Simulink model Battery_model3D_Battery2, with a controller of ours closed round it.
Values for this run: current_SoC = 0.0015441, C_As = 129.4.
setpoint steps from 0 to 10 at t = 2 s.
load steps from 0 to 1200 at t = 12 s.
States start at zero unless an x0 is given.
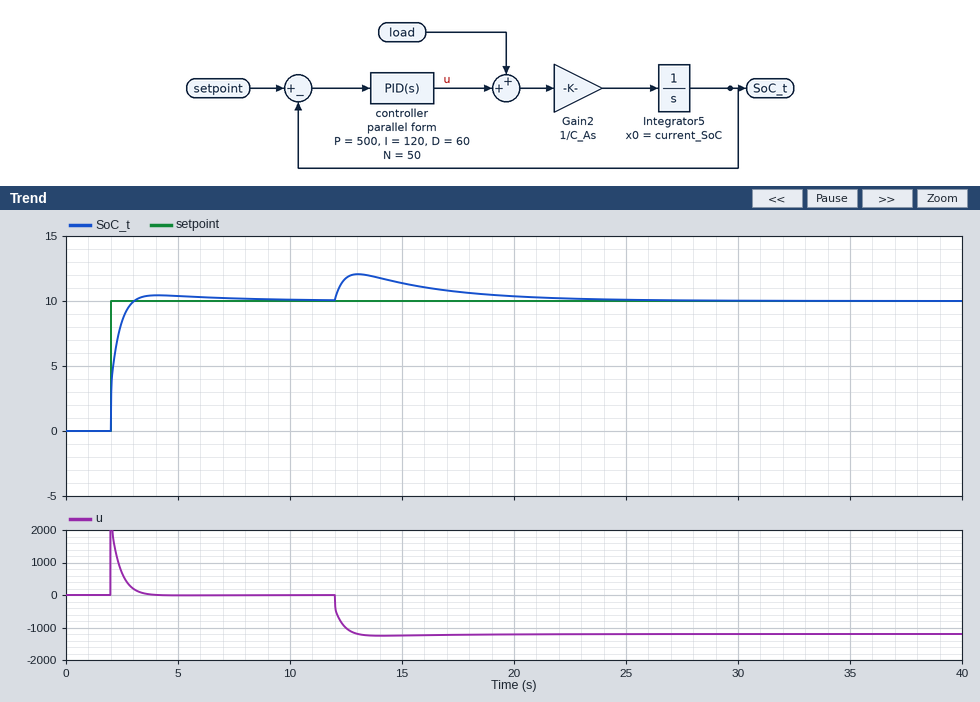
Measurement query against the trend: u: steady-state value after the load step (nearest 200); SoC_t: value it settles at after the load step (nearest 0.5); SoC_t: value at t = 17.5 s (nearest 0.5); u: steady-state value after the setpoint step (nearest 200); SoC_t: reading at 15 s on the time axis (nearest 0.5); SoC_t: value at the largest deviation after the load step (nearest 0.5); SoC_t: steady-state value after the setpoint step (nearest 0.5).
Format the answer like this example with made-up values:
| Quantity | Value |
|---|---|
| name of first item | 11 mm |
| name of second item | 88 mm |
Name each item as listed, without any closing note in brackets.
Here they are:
| Quantity | Value |
|---|---|
| u: steady-state value after the load step | -1200 |
| SoC_t: value it settles at after the load step | 10.0 |
| SoC_t: value at t = 17.5 s | 10.5 |
| u: steady-state value after the setpoint step | 0 |
| SoC_t: reading at 15 s on the time axis | 11.5 |
| SoC_t: value at the largest deviation after the load step | 12.0 |
| SoC_t: steady-state value after the setpoint step | 10.0 |
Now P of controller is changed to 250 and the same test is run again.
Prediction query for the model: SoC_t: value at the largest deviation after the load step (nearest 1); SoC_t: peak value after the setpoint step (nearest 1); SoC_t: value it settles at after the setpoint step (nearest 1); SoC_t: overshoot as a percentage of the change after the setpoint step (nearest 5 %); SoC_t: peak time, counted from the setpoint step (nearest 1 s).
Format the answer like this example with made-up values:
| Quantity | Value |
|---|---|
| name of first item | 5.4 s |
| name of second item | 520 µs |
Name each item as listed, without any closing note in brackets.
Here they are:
| Quantity | Value |
|---|---|
| SoC_t: value at the largest deviation after the load step | 13 |
| SoC_t: peak value after the setpoint step | 11 |
| SoC_t: value it settles at after the setpoint step | 10 |
| SoC_t: overshoot as a percentage of the change after the setpoint step | 10 % |
| SoC_t: peak time, counted from the setpoint step | 3 s |
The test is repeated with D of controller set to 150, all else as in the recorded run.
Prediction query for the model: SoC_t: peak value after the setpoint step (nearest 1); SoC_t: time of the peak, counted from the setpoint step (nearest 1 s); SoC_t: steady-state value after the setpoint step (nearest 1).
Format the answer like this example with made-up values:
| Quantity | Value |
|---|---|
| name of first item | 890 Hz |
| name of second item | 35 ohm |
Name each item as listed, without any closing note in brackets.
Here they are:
| Quantity | Value |
|---|---|
| SoC_t: peak value after the setpoint step | 10 |
| SoC_t: time of the peak, counted from the setpoint step | 3 s |
| SoC_t: steady-state value after the setpoint step | 10 |
